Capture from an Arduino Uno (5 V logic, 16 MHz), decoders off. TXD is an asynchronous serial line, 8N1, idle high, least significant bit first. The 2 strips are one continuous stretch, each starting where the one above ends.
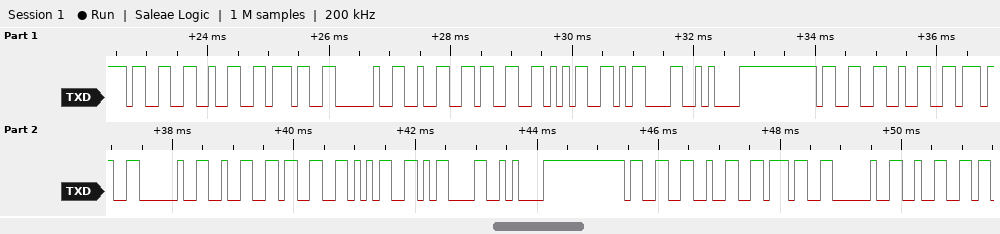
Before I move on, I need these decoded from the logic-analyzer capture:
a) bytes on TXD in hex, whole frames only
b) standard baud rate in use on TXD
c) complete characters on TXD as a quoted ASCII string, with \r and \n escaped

0x33 0x32 0x37 0x20 0x32 0x33 0x35 0x0D 0x0A 0x33 0x32 0x37 0x20 0x32 0x33 0x35 0x0D 0x0A 0x33 0x32 0x37 0x20 0x32
9600 baud
"327 235\r\n327 235\r\n327 2"
